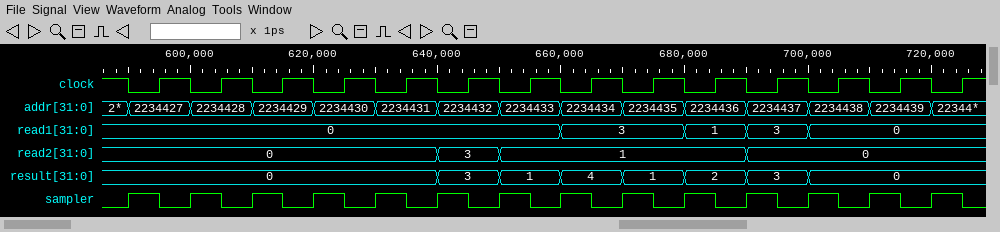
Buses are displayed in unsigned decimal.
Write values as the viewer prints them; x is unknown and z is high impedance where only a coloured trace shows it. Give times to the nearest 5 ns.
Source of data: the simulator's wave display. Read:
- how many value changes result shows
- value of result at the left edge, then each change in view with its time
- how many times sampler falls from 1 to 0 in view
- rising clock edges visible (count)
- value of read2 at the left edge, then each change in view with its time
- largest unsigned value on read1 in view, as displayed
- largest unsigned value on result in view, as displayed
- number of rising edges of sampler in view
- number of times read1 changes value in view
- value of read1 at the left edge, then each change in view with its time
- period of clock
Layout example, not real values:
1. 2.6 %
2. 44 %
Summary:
1. 7
2. 0, 3 at 640 ns, 1 at 650 ns, 4 at 660 ns, 1 at 670 ns, 2 at 680 ns, 3 at 690 ns, 0 at 700 ns
3. 14
4. 14
5. 0, 3 at 640 ns, 1 at 650 ns, 0 at 690 ns
6. 3
7. 4
8. 14
9. 4
10. 0, 3 at 660 ns, 1 at 680 ns, 3 at 690 ns, 0 at 700 ns
11. 10 ns
